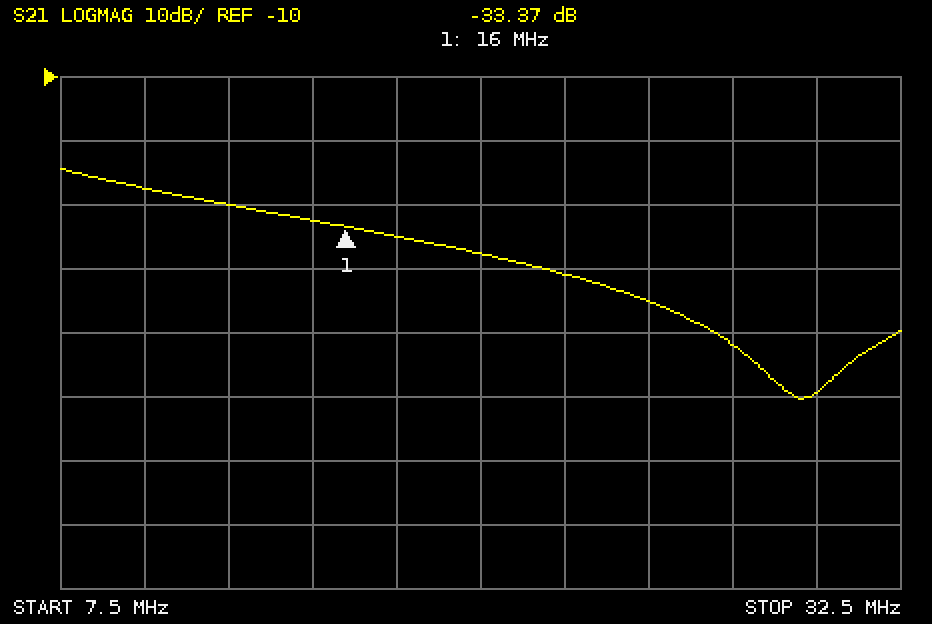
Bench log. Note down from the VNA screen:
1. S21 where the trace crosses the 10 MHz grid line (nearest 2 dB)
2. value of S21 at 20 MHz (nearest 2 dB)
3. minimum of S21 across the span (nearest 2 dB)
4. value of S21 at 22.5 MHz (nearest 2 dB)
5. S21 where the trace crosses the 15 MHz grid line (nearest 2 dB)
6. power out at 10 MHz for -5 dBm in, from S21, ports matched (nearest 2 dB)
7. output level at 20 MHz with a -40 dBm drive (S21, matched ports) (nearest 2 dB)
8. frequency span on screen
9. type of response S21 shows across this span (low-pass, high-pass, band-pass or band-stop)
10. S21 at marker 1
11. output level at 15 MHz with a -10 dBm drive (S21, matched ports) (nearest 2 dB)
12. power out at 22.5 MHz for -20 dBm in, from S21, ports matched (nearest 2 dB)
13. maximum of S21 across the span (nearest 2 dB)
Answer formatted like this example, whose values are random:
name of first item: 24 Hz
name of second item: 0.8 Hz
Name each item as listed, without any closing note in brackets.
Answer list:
S21 where the trace crosses the 10 MHz grid line: -28 dB
value of S21 at 20 MHz: -38 dB
minimum of S21 across the span: -60 dB
value of S21 at 22.5 MHz: -40 dB
S21 where the trace crosses the 15 MHz grid line: -32 dB
power out at 10 MHz for -5 dBm in, from S21, ports matched: -32 dBm
output level at 20 MHz with a -40 dBm drive (S21, matched ports): -78 dBm
frequency span on screen: 25 MHz
type of response S21 shows across this span: low-pass
S21 at marker 1: -33.37 dB
output level at 15 MHz with a -10 dBm drive (S21, matched ports): -42 dBm
power out at 22.5 MHz for -20 dBm in, from S21, ports matched: -60 dBm
maximum of S21 across the span: -24 dB
